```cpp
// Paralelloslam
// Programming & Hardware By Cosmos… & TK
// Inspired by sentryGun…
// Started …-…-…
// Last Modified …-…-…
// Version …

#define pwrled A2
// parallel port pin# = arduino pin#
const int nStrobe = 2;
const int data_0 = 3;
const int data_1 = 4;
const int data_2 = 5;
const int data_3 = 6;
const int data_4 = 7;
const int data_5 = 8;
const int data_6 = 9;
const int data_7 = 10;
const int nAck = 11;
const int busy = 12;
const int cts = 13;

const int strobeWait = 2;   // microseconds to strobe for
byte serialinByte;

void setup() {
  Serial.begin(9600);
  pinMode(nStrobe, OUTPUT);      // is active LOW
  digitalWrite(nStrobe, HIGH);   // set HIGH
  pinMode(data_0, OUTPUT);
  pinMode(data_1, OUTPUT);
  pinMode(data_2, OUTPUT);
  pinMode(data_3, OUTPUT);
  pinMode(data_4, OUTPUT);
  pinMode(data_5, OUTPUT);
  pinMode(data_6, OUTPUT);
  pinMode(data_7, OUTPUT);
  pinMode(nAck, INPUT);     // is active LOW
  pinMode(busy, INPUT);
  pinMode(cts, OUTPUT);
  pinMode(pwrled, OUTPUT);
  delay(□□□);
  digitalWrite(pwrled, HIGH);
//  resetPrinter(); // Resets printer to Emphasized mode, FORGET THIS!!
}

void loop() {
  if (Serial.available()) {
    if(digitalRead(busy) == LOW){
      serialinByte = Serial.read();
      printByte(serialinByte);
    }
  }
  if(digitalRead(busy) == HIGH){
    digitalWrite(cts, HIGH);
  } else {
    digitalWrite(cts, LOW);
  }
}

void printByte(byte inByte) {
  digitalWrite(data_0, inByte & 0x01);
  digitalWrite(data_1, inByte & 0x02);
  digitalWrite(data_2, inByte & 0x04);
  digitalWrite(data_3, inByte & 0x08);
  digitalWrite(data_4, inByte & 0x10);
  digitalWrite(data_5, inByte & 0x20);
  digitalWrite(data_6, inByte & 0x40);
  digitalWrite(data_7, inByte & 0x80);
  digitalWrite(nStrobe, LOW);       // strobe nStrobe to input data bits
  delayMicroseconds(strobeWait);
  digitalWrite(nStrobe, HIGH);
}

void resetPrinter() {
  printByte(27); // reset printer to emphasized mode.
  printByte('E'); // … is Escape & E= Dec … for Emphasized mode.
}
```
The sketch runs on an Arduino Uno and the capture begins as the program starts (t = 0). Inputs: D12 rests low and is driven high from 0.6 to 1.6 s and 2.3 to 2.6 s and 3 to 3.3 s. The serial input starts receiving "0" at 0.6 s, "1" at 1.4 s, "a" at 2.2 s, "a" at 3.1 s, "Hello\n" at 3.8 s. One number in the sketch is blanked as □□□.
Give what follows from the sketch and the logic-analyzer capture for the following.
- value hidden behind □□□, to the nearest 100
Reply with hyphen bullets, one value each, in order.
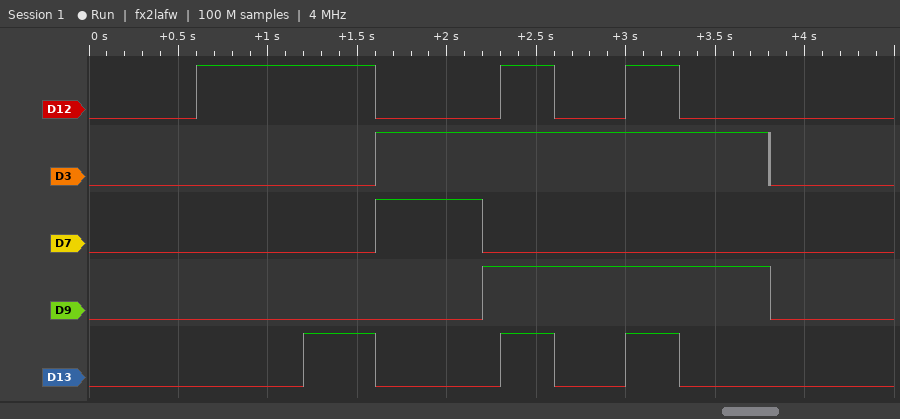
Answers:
- 1200
